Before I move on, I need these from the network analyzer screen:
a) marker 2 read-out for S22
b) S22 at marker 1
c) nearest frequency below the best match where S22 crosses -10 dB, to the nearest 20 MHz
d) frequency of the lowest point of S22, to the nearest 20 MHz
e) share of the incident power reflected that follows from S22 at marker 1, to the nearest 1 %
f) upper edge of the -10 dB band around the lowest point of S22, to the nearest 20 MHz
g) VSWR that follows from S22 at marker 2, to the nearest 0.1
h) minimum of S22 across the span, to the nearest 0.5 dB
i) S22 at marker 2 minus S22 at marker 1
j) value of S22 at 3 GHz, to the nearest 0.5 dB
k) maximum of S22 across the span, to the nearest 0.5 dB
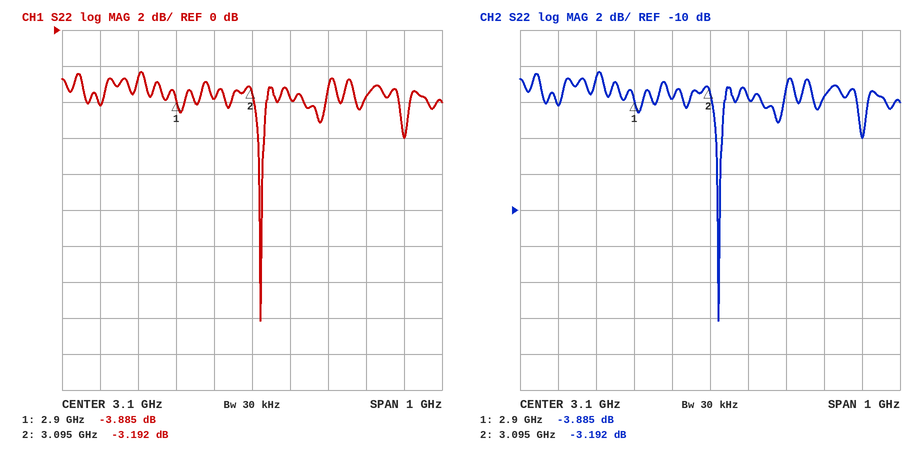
-3.192 dB
-3.885 dB
3.12 GHz
3.12 GHz
41 %
3.12 GHz
5.5
-16.0 dB
0.693 dB
-4.0 dB
-2.5 dB
